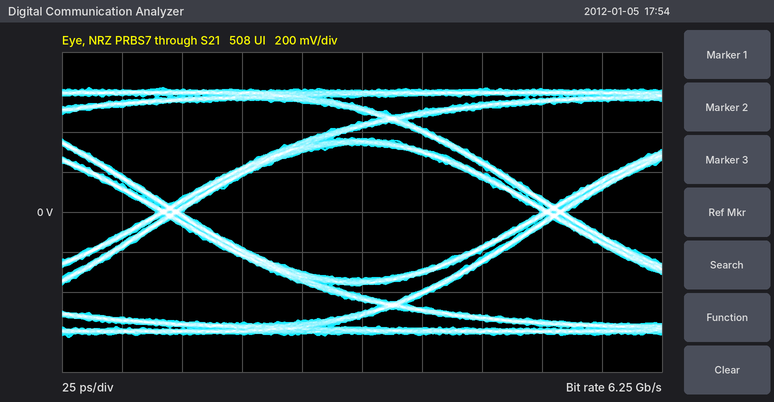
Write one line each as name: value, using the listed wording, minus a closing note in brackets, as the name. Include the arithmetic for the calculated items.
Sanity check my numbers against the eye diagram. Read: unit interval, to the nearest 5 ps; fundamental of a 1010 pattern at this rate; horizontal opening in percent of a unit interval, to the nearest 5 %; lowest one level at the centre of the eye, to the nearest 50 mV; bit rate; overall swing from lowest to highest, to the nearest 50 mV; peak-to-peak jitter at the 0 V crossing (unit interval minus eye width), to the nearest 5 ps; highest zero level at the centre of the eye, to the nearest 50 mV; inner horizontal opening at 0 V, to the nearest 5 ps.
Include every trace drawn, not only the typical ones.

unit interval, to the nearest 5 ps: 160 ps
fundamental of a 1010 pattern at this rate: 3.125 GHz
horizontal opening in percent of a unit interval, to the nearest 5 %: 150 ps / 160 ps ≈ 93.8 %, so 95 % to the nearest 5 %
lowest one level at the centre of the eye, to the nearest 50 mV: 350 mV
bit rate: 6.25 Gb/s
overall swing from lowest to highest, to the nearest 50 mV: 1.25 V
peak-to-peak jitter at the 0 V crossing (unit interval minus eye width), to the nearest 5 ps: 10 ps
highest zero level at the centre of the eye, to the nearest 50 mV: -350 mV
inner horizontal opening at 0 V, to the nearest 5 ps: 150 ps
